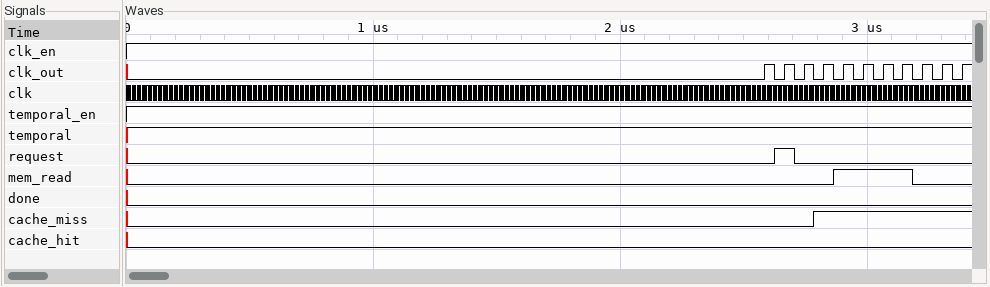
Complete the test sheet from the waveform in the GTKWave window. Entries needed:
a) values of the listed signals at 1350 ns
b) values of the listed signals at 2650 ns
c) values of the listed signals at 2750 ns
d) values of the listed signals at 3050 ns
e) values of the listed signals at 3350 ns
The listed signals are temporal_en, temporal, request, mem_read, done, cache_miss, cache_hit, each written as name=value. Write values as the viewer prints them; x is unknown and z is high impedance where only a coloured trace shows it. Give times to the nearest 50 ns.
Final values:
temporal_en=1, temporal=1, request=0, mem_read=0, done=0, cache_miss=0, cache_hit=0
temporal_en=1, temporal=1, request=1, mem_read=0, done=0, cache_miss=0, cache_hit=0
temporal_en=1, temporal=1, request=0, mem_read=0, done=0, cache_miss=0, cache_hit=0
temporal_en=1, temporal=1, request=0, mem_read=1, done=0, cache_miss=1, cache_hit=0
temporal_en=1, temporal=1, request=0, mem_read=0, done=0, cache_miss=1, cache_hit=0
